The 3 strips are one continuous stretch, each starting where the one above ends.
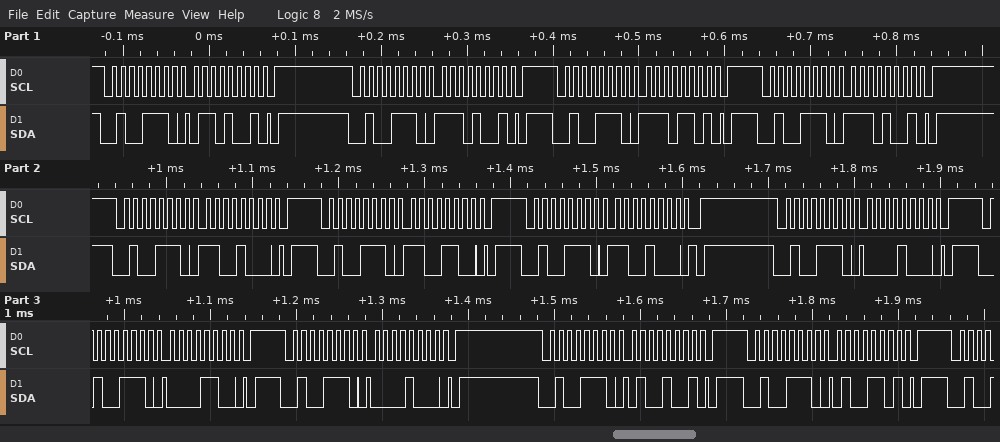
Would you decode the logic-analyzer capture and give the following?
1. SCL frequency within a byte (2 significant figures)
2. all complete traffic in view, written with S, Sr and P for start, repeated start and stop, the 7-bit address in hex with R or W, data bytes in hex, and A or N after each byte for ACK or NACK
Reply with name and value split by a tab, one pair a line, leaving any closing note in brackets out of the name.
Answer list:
SCL frequency within a byte	100 kHz
all complete traffic in view, written with S, Sr and P for start, repeated start and stop, the 7-bit address in hex with R or W, data bytes in hex, and A or N after each byte for ACK or NACK	S 27W A 69 A P S 27W A E9 A P S 27W A ED A P S 27W A E9 A P S 27W A C8 A P S 27W A CC A P S 27W A C8 A P S 27W A 08 A P S 27W A 0C A P S 27W A 08 A P S 27W A 49 A P S 27W A 4D A P
